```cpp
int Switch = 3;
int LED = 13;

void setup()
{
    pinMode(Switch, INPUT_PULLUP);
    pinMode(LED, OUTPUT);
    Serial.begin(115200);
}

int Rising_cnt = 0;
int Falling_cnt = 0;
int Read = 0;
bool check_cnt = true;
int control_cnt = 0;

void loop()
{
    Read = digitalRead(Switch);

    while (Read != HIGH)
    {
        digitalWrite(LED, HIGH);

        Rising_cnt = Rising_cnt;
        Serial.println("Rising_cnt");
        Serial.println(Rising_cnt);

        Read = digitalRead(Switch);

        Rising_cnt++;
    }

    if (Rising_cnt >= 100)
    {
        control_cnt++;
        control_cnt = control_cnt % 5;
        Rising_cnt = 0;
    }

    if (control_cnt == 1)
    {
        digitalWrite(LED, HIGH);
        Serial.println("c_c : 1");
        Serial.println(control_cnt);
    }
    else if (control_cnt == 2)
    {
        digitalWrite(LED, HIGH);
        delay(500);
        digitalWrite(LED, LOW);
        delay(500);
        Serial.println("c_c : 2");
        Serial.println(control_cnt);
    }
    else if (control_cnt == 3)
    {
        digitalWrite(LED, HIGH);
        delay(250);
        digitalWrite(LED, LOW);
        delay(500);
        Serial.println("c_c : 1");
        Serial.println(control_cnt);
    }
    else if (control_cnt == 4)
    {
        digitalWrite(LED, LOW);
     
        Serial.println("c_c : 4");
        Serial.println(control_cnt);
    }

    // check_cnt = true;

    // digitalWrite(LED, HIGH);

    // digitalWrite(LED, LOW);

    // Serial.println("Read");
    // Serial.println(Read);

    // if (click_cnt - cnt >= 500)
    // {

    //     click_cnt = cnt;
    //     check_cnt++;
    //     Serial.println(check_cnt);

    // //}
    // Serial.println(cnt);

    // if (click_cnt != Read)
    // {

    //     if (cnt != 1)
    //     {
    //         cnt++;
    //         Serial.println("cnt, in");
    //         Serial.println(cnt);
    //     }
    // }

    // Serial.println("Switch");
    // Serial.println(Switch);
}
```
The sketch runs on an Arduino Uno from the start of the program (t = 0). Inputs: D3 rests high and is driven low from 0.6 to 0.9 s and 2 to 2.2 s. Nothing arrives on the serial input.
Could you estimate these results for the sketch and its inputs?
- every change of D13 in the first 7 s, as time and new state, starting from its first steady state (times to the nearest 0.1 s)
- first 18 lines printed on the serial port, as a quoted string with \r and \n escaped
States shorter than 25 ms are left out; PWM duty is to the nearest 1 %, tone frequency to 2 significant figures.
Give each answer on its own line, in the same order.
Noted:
0 s low; 0.6 s high; 2.7 s low; 3.2 s high; 3.7 s low; 4.2 s high; 4.7 s low; 5.2 s high; 5.7 s low; 6.2 s high; 6.7 s low
"Rising_cnt\r\n0\r\nRising_cnt\r\n1\r\nRising_cnt\r\n2\r\nRising_cnt\r\n3\r\nRising_cnt\r\n4\r\nRising_cnt\r\n5\r\nRising_cnt\r\n6\r\nRising_cnt\r\n7\r\nRising_cnt\r\n8\r\n"
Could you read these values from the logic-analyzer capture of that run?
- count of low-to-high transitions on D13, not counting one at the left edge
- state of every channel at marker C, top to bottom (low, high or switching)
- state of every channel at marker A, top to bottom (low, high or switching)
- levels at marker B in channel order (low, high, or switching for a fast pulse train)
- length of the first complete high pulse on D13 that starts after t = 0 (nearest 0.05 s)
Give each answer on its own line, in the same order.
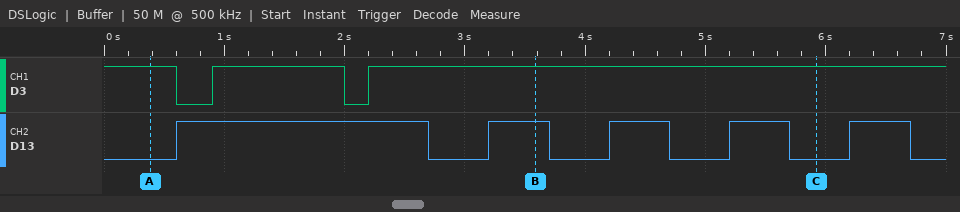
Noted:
5
D3 high, D13 low
D3 high, D13 low
D3 high, D13 high
2.10 s
